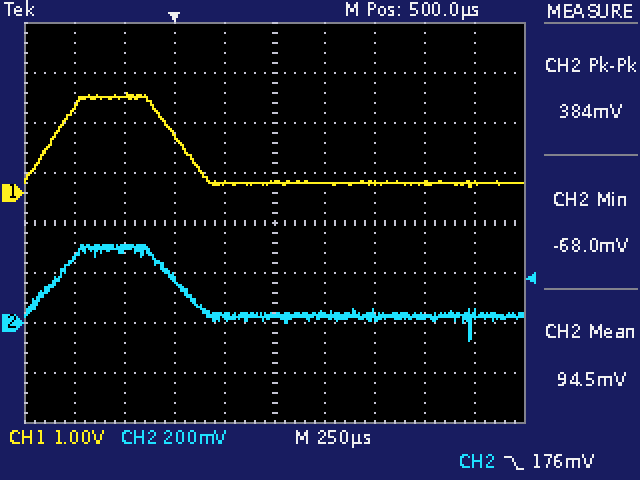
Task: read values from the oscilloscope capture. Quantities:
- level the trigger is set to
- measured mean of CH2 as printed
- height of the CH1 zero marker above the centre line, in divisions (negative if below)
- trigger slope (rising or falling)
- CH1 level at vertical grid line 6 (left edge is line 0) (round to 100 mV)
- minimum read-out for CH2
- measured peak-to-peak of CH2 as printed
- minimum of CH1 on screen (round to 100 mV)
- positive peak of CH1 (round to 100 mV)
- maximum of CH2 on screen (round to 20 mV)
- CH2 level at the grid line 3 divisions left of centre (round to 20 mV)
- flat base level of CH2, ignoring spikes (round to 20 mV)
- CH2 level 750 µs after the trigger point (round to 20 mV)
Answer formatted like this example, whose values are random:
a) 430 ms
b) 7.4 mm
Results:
a) 176 mV
b) 94.5 mV
c) +0.6 div
d) falling
e) 200 mV
f) -68.0 mV
g) 384 mV
h) 100 mV
i) 2.0 V
j) 320 mV
k) 300 mV
l) 20 mV
m) 40 mV
